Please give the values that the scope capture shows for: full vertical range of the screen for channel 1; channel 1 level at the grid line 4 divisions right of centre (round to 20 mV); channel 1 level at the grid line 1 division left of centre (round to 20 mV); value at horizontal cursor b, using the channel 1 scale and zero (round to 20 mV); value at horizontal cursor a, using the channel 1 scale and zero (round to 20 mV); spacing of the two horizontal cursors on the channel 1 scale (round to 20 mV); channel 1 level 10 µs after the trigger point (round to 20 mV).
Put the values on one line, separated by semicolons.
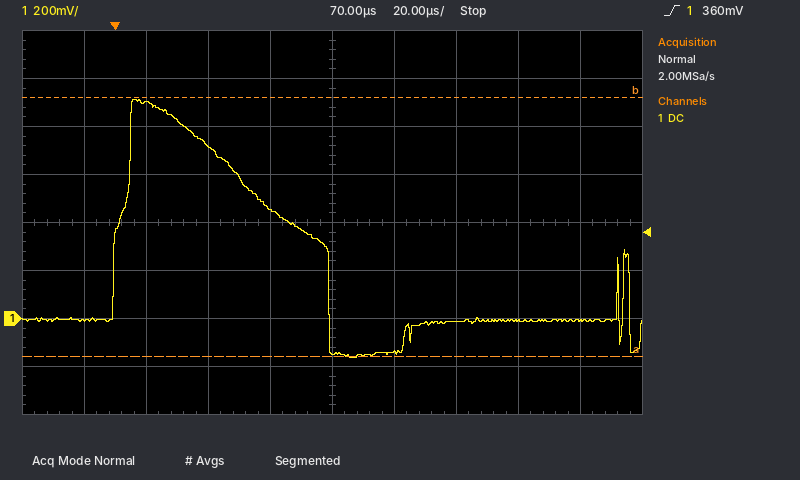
1.6 V; 0 mV; 460 mV; 920 mV; -160 mV; 1.08 V; 900 mV
